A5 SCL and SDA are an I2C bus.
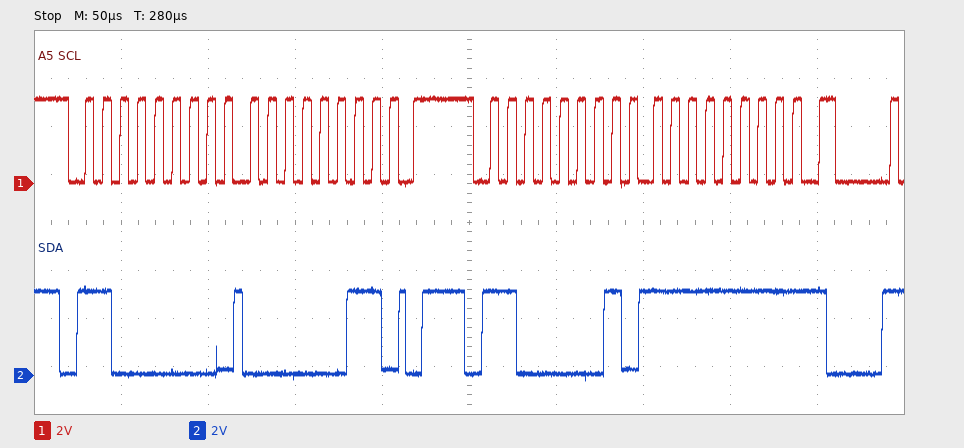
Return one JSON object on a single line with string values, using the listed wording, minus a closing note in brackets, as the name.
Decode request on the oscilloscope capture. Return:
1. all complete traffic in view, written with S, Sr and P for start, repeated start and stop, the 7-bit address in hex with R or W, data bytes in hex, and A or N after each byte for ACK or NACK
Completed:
{"all complete traffic in view, written with S, Sr and P for start, repeated start and stop, the 7-bit address in hex with R or W, data bytes in hex, and A or N after each byte for ACK or NACK": "S 60W A 03 A P S 60R A FF N"}
